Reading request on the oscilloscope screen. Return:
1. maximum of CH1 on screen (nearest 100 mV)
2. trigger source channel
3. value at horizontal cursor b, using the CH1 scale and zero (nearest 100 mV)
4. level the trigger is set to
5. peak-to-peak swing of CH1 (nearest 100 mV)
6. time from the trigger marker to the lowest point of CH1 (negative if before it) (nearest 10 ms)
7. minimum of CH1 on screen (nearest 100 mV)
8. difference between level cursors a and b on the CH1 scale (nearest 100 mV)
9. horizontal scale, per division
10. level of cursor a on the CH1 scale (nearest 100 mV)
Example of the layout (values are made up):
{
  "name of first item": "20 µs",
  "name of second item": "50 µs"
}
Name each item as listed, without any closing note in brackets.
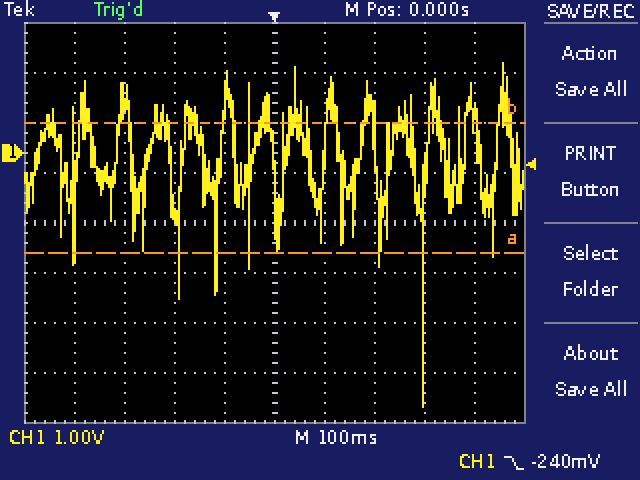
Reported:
{
  "maximum of CH1 on screen": "1.8 V",
  "trigger source channel": "CH1",
  "value at horizontal cursor b, using the CH1 scale and zero": "600 mV",
  "level the trigger is set to": "-240 mV",
  "peak-to-peak swing of CH1": "6.9 V",
  "time from the trigger marker to the lowest point of CH1 (negative if before it)": "+300 ms",
  "minimum of CH1 on screen": "-5.1 V",
  "difference between level cursors a and b on the CH1 scale": "2.6 V",
  "horizontal scale, per division": "100 ms",
  "level of cursor a on the CH1 scale": "-2.0 V"
}
